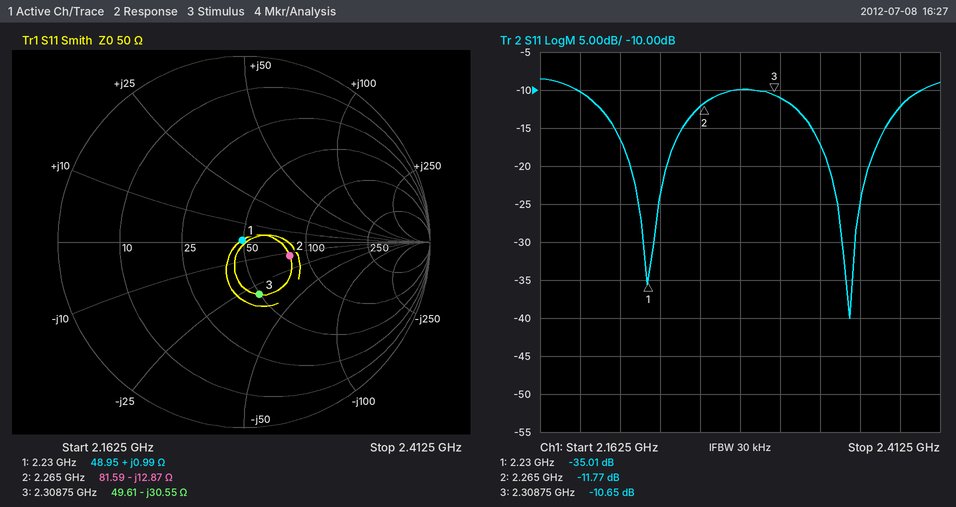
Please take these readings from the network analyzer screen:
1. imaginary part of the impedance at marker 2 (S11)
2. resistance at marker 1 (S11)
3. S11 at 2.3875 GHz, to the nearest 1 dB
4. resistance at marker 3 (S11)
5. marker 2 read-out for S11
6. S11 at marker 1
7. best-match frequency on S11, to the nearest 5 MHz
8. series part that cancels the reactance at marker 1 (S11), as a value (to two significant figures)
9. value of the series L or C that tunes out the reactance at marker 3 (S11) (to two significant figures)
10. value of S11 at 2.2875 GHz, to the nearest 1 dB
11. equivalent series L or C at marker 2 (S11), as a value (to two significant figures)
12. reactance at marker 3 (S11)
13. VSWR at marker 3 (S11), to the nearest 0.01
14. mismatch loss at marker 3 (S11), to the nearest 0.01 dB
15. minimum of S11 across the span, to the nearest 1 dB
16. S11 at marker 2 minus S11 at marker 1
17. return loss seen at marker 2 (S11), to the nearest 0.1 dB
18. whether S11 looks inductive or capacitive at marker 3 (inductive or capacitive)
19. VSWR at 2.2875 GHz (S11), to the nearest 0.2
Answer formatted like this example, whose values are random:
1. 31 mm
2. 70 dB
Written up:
1. -12.87 Ω
2. 48.95 Ω
3. -12 dB
4. 49.61 Ω
5. -11.77 dB
6. -35.01 dB
7. 2.355 GHz
8. 72 pF
9. 2.1 nH
10. -10 dB
11. 5.5 pF
12. -30.55 Ω
13. 1.83
14. 0.39 dB
15. -40 dB
16. 23.24 dB
17. 11.8 dB
18. capacitive
19. 2.0
